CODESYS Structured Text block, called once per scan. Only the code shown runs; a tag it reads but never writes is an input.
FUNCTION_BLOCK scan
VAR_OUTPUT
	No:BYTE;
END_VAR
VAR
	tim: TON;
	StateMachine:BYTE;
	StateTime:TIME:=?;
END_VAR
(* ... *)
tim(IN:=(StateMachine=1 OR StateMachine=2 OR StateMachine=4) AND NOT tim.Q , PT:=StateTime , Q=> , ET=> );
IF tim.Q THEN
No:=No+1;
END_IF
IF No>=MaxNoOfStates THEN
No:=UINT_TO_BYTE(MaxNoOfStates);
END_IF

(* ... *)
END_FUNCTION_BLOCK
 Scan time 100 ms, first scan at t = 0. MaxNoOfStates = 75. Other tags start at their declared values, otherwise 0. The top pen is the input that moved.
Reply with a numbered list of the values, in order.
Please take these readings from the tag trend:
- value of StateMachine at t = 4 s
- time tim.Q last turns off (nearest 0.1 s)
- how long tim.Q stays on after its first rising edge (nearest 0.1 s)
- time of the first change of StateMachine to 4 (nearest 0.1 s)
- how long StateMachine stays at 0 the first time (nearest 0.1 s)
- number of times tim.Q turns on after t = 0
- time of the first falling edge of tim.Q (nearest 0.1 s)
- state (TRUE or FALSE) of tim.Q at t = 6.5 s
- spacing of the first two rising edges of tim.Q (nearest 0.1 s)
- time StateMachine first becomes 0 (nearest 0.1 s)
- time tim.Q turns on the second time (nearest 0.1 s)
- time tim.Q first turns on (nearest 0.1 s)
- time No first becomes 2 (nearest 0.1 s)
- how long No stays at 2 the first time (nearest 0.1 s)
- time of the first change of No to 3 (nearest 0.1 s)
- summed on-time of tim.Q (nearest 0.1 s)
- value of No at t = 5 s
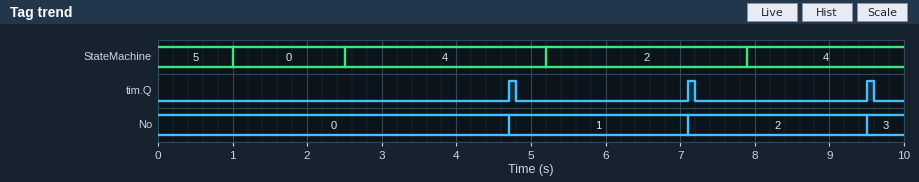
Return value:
1. 4
2. 9.6 s
3. 0.1 s
4. 2.5 s
5. 1.5 s
6. 3
7. 4.8 s
8. FALSE
9. 2.4 s
10. 1.0 s
11. 7.1 s
12. 4.7 s
13. 7.1 s
14. 2.4 s
15. 9.5 s
16. 0.3 s
17. 1
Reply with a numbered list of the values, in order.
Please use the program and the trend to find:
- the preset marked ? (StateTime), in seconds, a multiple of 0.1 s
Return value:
1. 2.2 s
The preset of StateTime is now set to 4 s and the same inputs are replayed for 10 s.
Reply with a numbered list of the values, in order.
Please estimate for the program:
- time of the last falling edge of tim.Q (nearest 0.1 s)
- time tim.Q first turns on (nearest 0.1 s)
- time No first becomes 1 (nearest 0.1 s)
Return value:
1. 6.6 s
2. 6.5 s
3. 6.5 s
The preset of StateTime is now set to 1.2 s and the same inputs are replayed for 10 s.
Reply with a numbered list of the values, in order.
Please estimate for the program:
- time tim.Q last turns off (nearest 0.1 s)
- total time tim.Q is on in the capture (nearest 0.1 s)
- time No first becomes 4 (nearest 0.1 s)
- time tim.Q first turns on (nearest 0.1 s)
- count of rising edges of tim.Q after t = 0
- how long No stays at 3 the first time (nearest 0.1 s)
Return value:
1. 9.4 s
2. 0.5 s
3. 7.9 s
4. 3.7 s
5. 5
6. 1.4 s
